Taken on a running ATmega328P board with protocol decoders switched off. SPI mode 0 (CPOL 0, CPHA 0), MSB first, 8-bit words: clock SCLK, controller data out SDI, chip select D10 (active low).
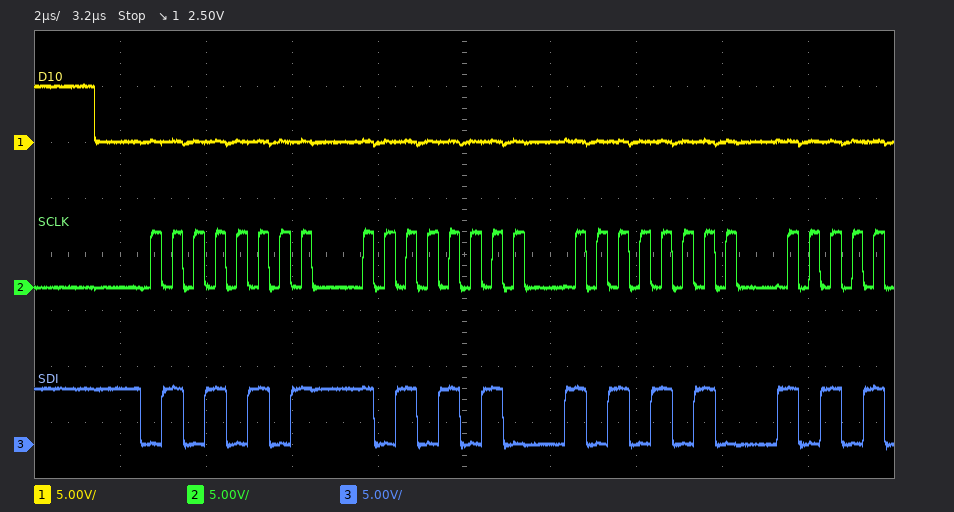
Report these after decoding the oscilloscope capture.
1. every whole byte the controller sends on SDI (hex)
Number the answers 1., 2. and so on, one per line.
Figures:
1. 55 AA AA
